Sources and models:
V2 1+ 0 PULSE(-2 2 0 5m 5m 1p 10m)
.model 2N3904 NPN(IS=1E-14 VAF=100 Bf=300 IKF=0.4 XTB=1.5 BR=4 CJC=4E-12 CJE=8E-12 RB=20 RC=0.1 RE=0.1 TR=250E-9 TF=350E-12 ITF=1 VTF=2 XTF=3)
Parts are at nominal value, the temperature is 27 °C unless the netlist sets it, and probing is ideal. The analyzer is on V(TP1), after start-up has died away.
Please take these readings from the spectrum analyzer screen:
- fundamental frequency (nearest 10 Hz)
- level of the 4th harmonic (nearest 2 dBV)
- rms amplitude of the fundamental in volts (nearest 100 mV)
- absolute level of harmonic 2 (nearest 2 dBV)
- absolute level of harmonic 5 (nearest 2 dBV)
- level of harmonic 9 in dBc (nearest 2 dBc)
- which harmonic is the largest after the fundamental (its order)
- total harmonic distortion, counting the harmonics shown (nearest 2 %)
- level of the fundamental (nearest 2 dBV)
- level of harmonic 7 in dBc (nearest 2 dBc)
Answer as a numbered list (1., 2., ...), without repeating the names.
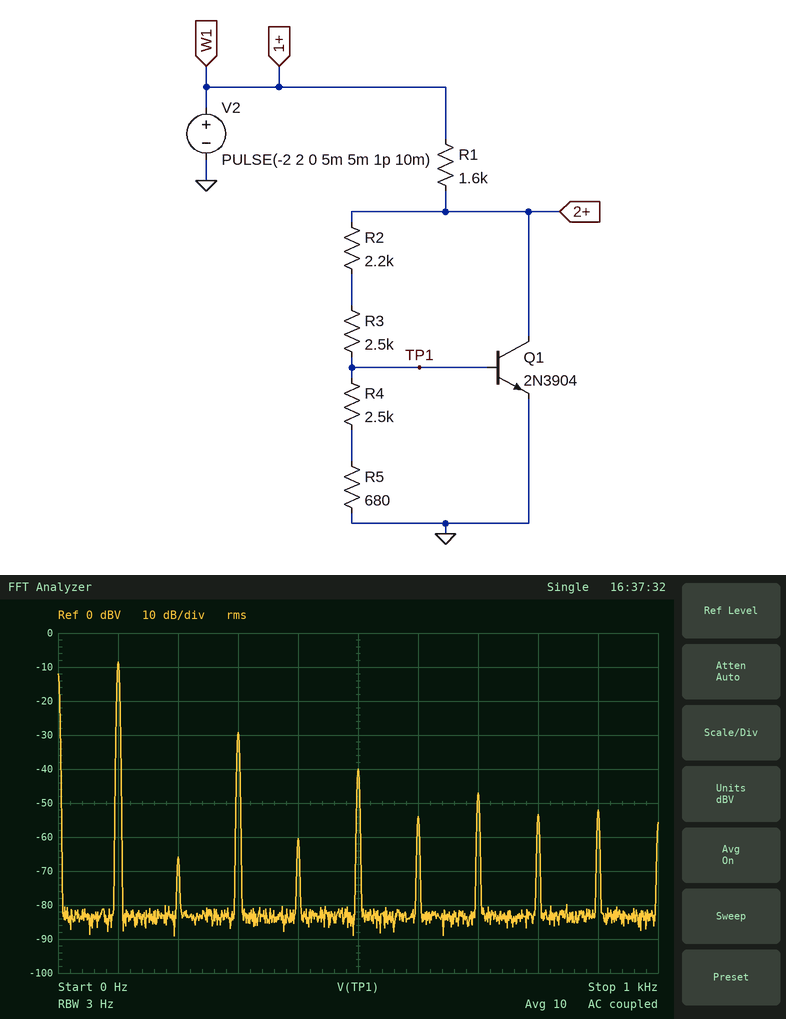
1. 100 Hz
2. -60 dBV
3. 400 mV
4. -66 dBV
5. -40 dBV
6. -44 dBc
7. 3
8. 10 %
9. -8 dBV
10. -38 dBc
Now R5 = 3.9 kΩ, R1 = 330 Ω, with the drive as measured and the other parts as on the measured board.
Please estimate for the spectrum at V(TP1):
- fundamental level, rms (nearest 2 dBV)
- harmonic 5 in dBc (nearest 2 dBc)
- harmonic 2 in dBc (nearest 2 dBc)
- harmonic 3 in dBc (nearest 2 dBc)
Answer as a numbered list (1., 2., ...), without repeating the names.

1. -4 dBV
2. -34 dBc
3. -18 dBc
4. -24 dBc
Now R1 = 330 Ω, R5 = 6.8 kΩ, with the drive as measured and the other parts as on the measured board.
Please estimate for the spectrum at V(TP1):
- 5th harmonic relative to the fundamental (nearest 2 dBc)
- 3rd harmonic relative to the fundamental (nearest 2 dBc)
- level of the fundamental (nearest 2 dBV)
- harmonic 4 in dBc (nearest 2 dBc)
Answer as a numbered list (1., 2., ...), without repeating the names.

1. -36 dBc
2. -30 dBc
3. -4 dBV
4. -24 dBc
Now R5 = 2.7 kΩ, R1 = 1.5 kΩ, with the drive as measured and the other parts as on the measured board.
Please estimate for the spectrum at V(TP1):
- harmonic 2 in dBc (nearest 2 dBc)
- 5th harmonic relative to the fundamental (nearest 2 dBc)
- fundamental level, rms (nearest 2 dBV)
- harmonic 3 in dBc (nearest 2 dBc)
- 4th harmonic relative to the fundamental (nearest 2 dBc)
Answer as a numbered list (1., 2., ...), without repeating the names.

1. -24 dBc
2. -44 dBc
3. -6 dBV
4. -24 dBc
5. -28 dBc
